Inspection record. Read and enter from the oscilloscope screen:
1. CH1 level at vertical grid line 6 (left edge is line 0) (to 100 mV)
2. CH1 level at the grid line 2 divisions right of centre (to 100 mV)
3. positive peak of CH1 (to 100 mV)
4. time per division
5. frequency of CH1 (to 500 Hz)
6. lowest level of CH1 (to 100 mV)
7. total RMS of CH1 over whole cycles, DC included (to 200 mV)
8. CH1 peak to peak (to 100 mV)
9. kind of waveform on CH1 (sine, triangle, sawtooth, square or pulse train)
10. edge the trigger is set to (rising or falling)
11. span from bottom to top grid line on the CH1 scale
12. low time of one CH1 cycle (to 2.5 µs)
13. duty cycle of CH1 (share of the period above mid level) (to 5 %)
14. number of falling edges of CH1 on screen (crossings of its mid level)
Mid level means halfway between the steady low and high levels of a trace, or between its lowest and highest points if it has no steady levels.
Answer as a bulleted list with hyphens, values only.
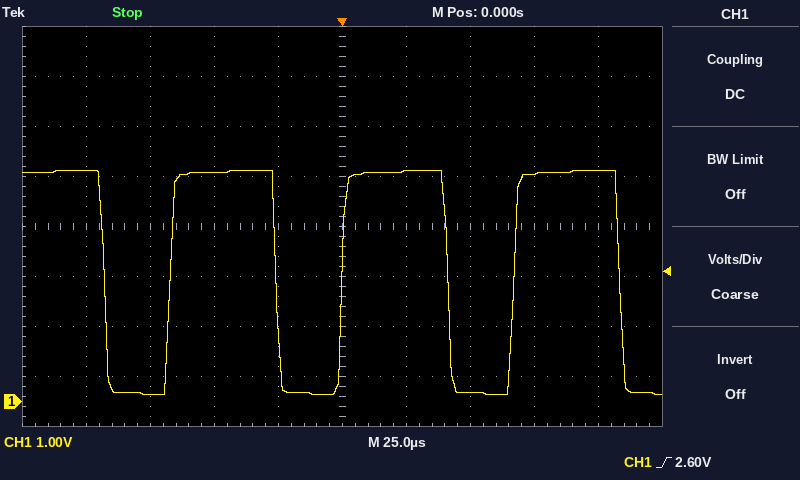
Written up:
- 4.6 V
- 200 mV
- 4.6 V
- 25 µs
- 15.0 kHz
- 100 mV
- 3.6 V
- 4.5 V
- pulse train
- rising
- 8 V
- 25.0 µs
- 60 %
- 4
